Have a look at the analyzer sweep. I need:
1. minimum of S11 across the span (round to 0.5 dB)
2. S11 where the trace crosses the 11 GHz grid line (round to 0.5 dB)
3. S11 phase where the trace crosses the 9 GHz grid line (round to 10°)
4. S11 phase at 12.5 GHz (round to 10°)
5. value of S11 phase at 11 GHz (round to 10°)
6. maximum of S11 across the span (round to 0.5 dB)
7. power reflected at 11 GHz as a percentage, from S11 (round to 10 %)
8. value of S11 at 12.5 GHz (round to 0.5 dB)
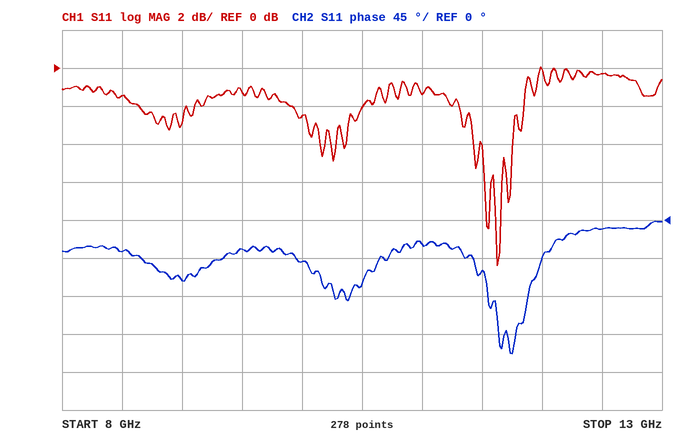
-10.5 dB
-1.5 dB
-70°
-10°
-30°
0.0 dB
70 %
-0.5 dB
